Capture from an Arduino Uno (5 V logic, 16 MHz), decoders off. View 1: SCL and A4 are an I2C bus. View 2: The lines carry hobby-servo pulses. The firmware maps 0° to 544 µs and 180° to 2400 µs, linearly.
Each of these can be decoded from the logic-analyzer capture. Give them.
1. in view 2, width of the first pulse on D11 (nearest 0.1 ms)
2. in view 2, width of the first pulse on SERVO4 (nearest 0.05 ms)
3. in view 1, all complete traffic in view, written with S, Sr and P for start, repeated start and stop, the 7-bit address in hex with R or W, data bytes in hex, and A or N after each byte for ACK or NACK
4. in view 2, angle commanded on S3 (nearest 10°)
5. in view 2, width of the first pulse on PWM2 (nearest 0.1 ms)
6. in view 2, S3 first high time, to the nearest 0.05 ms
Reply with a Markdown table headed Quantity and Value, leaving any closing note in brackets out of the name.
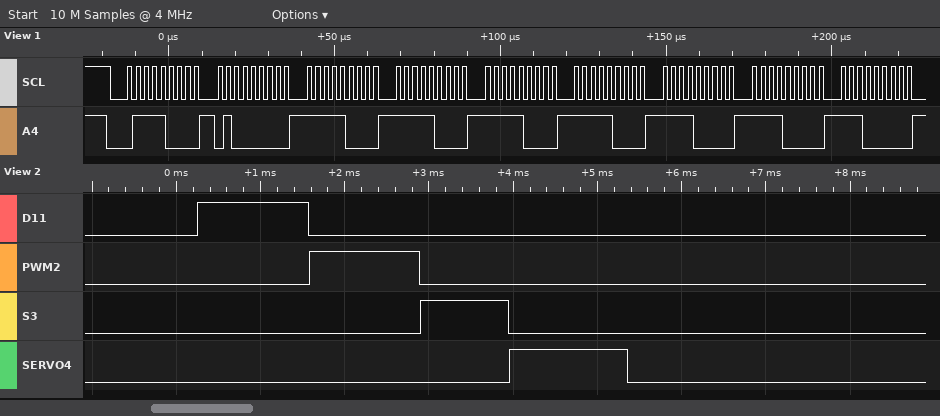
| Quantity | Value |
|---|---|
| in view 2, width of the first pulse on D11 | 1.3 ms |
| in view 2, width of the first pulse on SERVO4 | 1.40 ms |
| in view 1, all complete traffic in view, written with S, Sr and P for start, repeated start and stop, the 7-bit address in hex with R or W, data bytes in hex, and A or N after each byte for ACK or NACK | S 3CW A 40 A F8 A F8 A F8 A F8 A F0 A F0 A E0 A |
| in view 2, angle commanded on S3 | 50° |
| in view 2, width of the first pulse on PWM2 | 1.3 ms |
| in view 2, S3 first high time, to the nearest 0.05 ms | 1.05 ms |
